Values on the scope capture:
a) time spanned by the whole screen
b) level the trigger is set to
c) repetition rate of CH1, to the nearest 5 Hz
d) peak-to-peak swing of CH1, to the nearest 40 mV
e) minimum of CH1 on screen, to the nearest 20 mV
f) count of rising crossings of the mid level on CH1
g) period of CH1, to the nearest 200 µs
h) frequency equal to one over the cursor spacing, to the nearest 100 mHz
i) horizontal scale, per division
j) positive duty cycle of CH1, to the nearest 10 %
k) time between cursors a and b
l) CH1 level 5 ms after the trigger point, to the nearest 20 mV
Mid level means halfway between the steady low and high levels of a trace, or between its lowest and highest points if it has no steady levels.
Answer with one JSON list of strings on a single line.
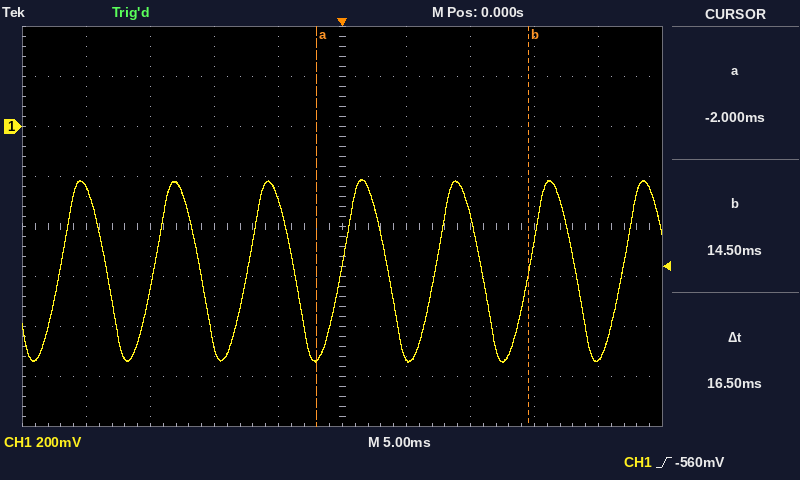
["50 ms", "-560 mV", "135 Hz", "720 mV", "-940 mV", "7", "7.4 ms", "60.6 Hz", "5 ms", "50 %", "16.5 ms", "-920 mV"]
